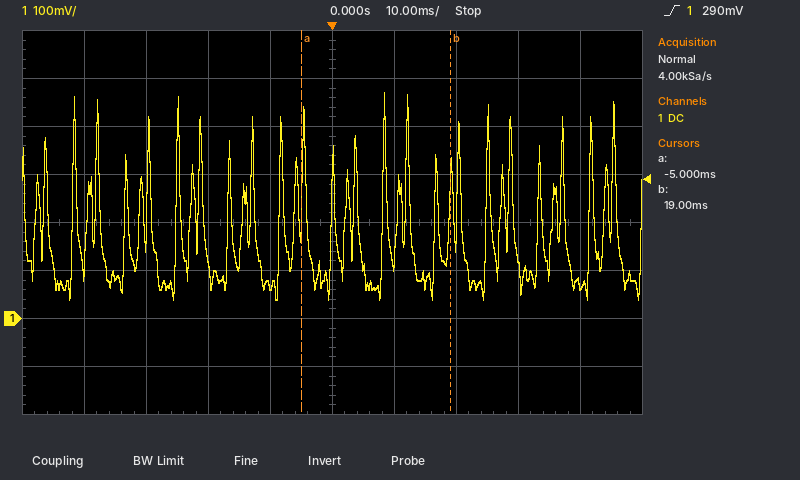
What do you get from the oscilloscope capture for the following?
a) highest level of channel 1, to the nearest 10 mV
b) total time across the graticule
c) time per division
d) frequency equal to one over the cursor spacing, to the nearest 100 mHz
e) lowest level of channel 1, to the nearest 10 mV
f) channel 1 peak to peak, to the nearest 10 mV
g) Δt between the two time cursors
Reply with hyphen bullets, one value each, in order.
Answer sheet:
- 470 mV
- 100 ms
- 10 ms
- 41.7 Hz
- 40 mV
- 430 mV
- 24 ms
